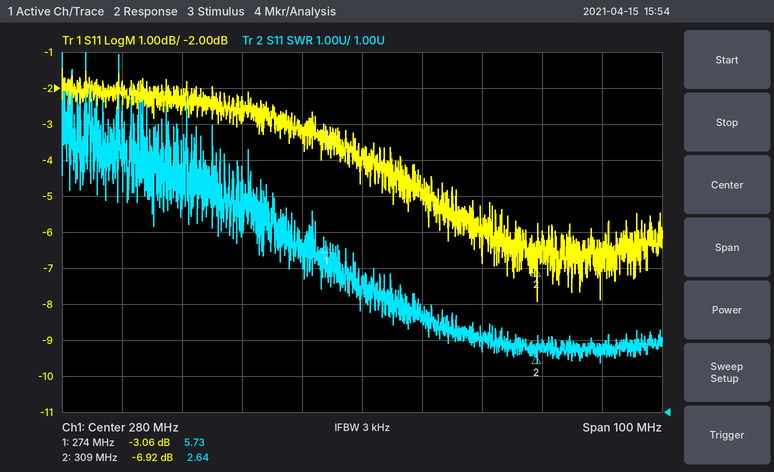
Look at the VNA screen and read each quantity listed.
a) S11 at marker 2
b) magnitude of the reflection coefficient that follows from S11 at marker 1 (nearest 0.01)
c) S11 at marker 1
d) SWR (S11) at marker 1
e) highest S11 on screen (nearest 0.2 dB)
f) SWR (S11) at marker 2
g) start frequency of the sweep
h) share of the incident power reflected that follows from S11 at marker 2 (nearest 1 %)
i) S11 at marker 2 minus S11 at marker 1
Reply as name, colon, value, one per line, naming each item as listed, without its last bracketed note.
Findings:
S11 at marker 2: -6.92 dB
magnitude of the reflection coefficient that follows from S11 at marker 1: 0.70
S11 at marker 1: -3.06 dB
SWR (S11) at marker 1: 5.73
highest S11 on screen: -1.4 dB
SWR (S11) at marker 2: 2.64
start frequency of the sweep: 230 MHz
share of the incident power reflected that follows from S11 at marker 2: 20 %
S11 at marker 2 minus S11 at marker 1: -3.86 dB
